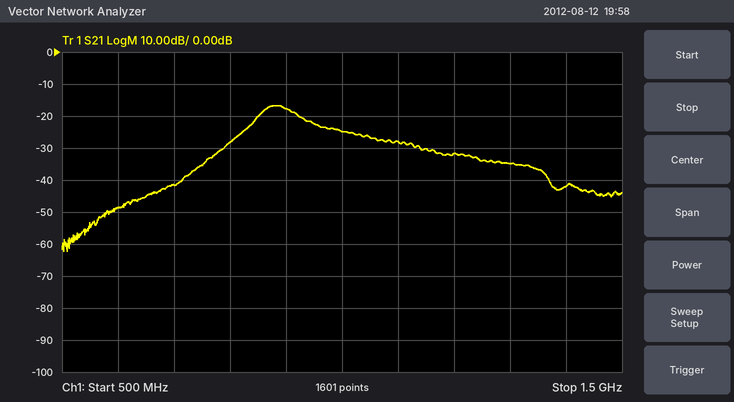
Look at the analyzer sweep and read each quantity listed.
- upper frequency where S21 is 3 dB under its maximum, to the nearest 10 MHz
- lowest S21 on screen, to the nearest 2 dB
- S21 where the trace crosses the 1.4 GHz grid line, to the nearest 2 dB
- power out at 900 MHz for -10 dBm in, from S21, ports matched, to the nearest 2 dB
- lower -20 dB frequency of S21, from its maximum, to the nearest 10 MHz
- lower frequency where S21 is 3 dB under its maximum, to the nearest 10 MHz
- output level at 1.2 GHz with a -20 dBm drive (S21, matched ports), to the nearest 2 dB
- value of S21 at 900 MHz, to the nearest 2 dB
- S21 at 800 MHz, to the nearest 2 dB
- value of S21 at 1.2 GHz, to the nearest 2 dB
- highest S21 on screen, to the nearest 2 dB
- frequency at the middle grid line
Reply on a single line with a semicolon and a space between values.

920 MHz; -62 dB; -42 dB; -28 dBm; 740 MHz; 850 MHz; -52 dBm; -18 dB; -28 dB; -32 dB; -16 dB; 1 GHz
